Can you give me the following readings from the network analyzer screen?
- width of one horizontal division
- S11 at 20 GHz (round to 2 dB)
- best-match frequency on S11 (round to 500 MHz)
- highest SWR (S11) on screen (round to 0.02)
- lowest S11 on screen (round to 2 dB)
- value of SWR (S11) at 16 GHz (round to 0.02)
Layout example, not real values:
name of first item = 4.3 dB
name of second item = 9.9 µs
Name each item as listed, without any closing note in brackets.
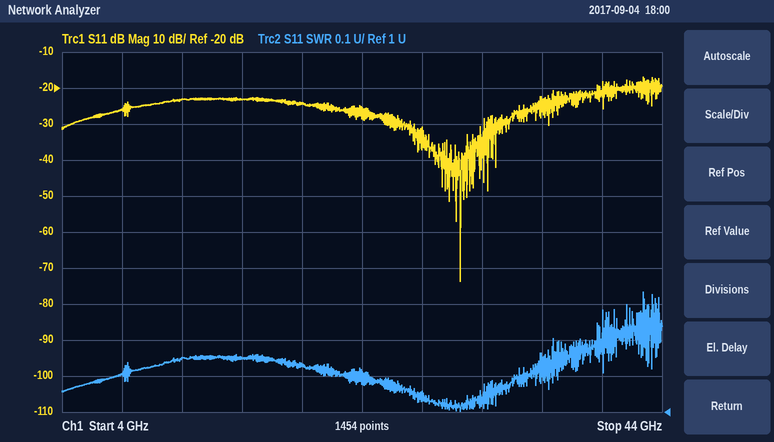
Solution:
width of one horizontal division = 4 GHz
S11 at 20 GHz = -24 dB
best-match frequency on S11 = 30.5 GHz
highest SWR (S11) on screen = 1.34
lowest S11 on screen = -74 dB
value of SWR (S11) at 16 GHz = 1.14
